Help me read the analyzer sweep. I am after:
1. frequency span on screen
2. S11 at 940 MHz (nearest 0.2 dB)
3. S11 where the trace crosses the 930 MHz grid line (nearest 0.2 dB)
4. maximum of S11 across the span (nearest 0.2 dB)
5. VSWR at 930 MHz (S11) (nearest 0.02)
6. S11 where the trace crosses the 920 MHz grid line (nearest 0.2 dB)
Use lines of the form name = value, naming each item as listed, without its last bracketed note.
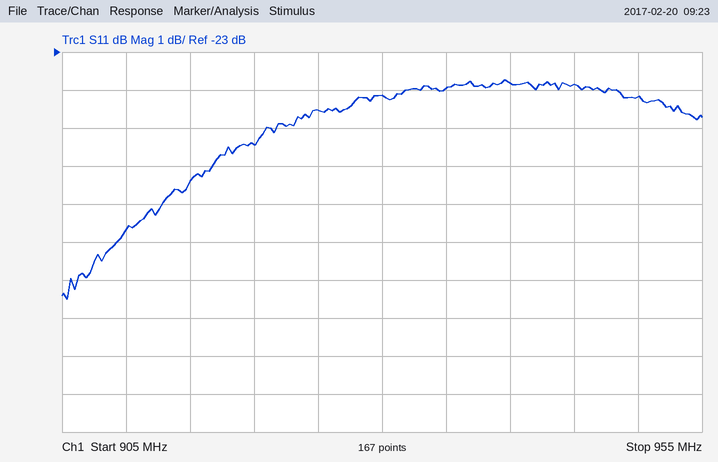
frequency span on screen = 50 MHz
S11 at 940 MHz = -23.8 dB
S11 where the trace crosses the 930 MHz grid line = -24.2 dB
maximum of S11 across the span = -23.8 dB
VSWR at 930 MHz (S11) = 1.14
S11 where the trace crosses the 920 MHz grid line = -25.4 dB
